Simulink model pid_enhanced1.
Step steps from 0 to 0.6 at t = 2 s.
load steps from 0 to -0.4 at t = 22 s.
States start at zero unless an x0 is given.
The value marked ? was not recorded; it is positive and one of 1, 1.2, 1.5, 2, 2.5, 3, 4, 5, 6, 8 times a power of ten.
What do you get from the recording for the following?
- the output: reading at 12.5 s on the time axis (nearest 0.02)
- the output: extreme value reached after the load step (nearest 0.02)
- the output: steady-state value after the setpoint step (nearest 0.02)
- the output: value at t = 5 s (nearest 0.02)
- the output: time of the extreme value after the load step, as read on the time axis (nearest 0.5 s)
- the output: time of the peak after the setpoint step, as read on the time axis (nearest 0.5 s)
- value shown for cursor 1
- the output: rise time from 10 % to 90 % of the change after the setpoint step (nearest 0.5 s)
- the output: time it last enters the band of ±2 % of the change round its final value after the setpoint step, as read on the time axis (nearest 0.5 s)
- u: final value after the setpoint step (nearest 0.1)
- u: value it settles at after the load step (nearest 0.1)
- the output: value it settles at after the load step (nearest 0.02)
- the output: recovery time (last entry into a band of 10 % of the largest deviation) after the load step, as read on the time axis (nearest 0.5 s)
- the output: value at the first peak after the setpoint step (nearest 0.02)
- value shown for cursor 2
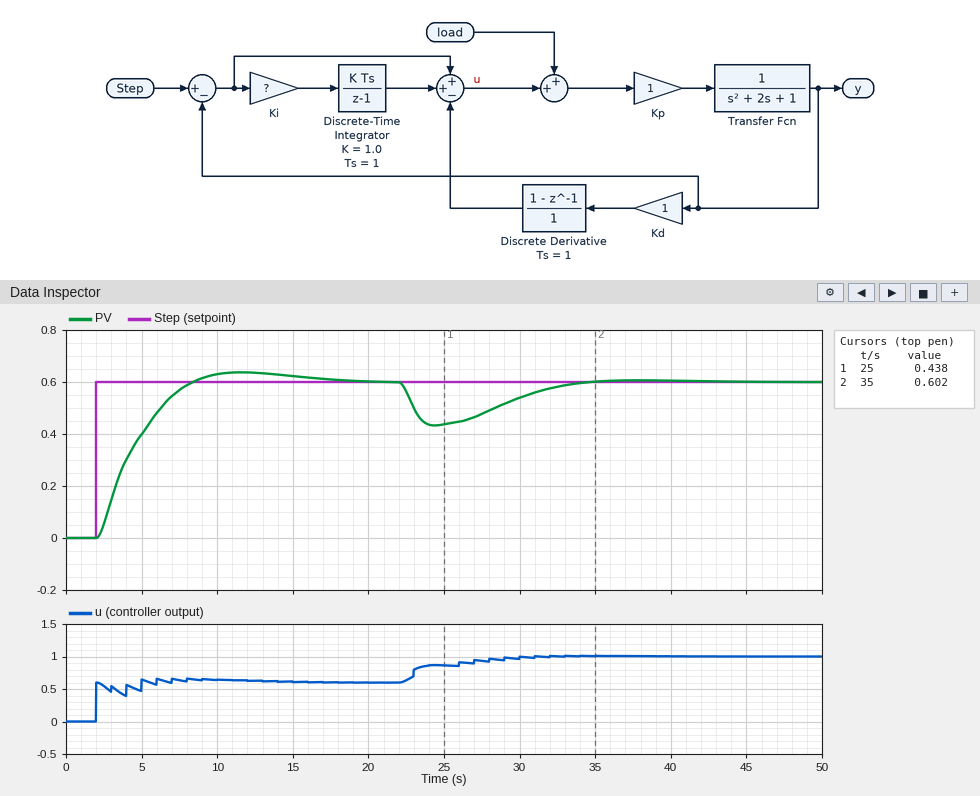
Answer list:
0.64
0.44
0.60
0.40
24.5 s
11.5 s
0.438
4.5 s
17.0 s
0.6
1.0
0.60
32.5 s
0.64
0.602
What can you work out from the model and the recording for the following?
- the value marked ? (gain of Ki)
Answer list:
0.4
